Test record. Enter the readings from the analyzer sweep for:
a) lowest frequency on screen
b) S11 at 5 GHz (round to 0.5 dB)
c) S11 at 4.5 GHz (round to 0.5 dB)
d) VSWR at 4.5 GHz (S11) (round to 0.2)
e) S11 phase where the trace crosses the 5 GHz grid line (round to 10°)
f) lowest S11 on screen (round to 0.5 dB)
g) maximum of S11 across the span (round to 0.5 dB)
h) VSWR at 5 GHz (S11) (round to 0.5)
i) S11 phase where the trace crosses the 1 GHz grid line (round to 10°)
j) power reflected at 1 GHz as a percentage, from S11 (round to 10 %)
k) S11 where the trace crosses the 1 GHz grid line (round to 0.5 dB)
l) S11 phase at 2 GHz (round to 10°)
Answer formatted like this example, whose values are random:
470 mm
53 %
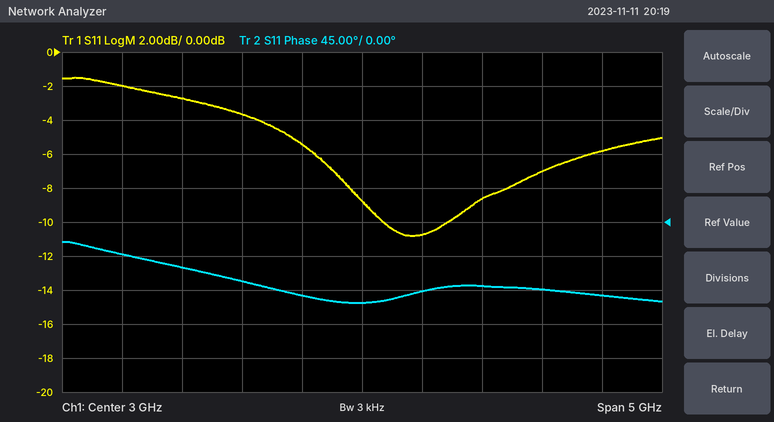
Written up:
500 MHz
-6.0 dB
-7.0 dB
2.6
-100°
-11.0 dB
-1.5 dB
3.0
-40°
60 %
-2.0 dB
-80°
